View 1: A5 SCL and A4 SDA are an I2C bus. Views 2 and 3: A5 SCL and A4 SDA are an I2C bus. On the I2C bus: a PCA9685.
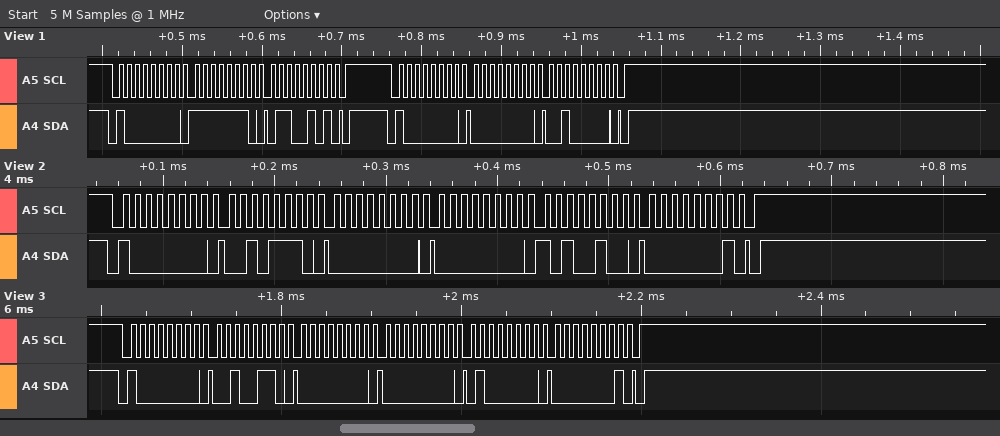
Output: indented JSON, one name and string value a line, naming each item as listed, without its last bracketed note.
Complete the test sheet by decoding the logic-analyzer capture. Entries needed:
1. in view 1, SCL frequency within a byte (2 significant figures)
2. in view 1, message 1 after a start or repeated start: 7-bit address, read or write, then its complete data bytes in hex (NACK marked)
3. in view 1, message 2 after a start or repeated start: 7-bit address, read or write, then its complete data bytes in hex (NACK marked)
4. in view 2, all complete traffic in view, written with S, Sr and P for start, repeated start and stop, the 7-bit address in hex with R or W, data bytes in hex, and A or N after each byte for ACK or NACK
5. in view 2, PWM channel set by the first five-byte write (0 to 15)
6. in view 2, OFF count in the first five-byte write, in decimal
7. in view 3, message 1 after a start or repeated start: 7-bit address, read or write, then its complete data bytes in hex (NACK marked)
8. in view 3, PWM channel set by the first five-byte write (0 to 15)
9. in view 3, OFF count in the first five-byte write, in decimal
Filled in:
{
  "in view 1, SCL frequency within a byte": "100 kHz",
  "in view 1, message 1 after a start or repeated start: 7-bit address, read or write, then its complete data bytes in hex": "0x40 write: FE 65",
  "in view 1, message 2 after a start or repeated start: 7-bit address, read or write, then its complete data bytes in hex": "0x40 write: 00 20",
  "in view 2, all complete traffic in view, written with S, Sr and P for start, repeated start and stop, the 7-bit address in hex with R or W, data bytes in hex, and A or N after each byte for ACK or NACK": "S 40W A 2E A 00 A 00 A A4 A 01 A P",
  "in view 2, PWM channel set by the first five-byte write": "10",
  "in view 2, OFF count in the first five-byte write, in decimal": "420",
  "in view 3, message 1 after a start or repeated start: 7-bit address, read or write, then its complete data bytes in hex": "0x40 write: 26 00 00 40 01",
  "in view 3, PWM channel set by the first five-byte write": "8",
  "in view 3, OFF count in the first five-byte write, in decimal": "320"
}
